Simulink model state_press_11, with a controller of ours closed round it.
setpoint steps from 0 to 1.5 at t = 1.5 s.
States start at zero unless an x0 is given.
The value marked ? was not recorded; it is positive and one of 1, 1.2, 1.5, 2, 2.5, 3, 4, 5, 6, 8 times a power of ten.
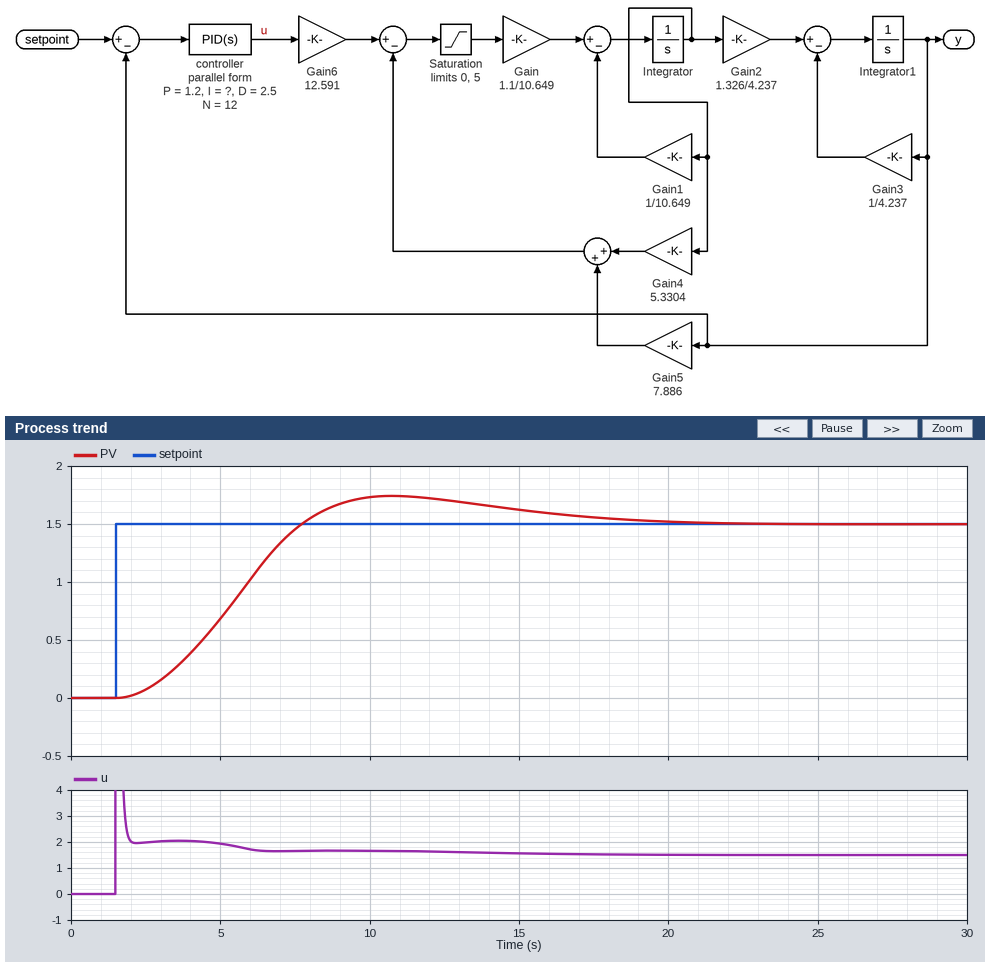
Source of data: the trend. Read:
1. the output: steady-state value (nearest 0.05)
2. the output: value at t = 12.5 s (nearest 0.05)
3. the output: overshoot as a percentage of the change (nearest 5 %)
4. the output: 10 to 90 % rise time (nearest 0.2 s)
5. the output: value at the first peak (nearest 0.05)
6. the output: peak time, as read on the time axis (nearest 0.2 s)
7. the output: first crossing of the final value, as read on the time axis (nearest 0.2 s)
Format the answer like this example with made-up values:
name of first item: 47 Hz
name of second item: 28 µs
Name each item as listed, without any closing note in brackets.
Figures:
the output: steady-state value: 1.50
the output: value at t = 12.5 s: 1.70
the output: overshoot as a percentage of the change: 15 %
the output: 10 to 90 % rise time: 4.0 s
the output: value at the first peak: 1.75
the output: peak time, as read on the time axis: 10.8 s
the output: first crossing of the final value, as read on the time axis: 7.8 s
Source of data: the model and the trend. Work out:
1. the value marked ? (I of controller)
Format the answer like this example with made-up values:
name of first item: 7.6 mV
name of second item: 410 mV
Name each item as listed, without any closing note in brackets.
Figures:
the value marked ?: 0.4
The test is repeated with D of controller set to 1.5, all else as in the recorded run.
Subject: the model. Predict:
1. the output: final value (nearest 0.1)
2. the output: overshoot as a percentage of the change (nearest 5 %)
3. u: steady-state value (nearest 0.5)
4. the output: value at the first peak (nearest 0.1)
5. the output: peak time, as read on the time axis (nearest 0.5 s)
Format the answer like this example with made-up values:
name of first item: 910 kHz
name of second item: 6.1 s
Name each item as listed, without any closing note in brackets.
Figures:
the output: final value: 1.5
the output: overshoot as a percentage of the change: 25 %
u: steady-state value: 1.5
the output: value at the first peak: 1.9
the output: peak time, as read on the time axis: 11.0 s
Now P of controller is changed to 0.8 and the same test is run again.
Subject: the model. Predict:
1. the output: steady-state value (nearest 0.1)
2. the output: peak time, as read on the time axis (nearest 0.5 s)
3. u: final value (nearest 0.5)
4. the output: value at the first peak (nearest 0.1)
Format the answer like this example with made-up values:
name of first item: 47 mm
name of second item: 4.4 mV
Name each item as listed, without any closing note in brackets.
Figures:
the output: steady-state value: 1.5
the output: peak time, as read on the time axis: 11.5 s
u: final value: 1.5
the output: value at the first peak: 1.8
